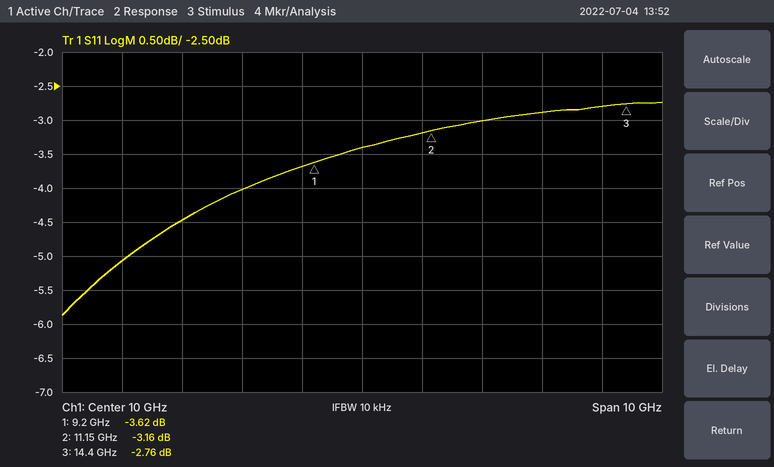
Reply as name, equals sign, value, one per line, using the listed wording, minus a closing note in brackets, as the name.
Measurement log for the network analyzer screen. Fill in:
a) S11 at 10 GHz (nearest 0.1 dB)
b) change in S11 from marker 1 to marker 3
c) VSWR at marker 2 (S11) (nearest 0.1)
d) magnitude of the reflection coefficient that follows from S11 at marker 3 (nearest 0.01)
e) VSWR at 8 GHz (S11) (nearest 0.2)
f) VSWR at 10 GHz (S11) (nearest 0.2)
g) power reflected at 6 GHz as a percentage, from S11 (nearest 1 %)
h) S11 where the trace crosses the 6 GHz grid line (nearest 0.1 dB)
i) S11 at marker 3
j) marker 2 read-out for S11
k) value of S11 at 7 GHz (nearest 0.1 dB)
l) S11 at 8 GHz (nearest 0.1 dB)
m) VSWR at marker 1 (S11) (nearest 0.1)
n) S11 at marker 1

S11 at 10 GHz = -3.4 dB
change in S11 from marker 1 to marker 3 = 0.86 dB
VSWR at marker 2 (S11) = 5.6
magnitude of the reflection coefficient that follows from S11 at marker 3 = 0.73
VSWR at 8 GHz (S11) = 4.4
VSWR at 10 GHz (S11) = 5.2
power reflected at 6 GHz as a percentage, from S11 = 31 %
S11 where the trace crosses the 6 GHz grid line = -5.1 dB
S11 at marker 3 = -2.76 dB
marker 2 read-out for S11 = -3.16 dB
value of S11 at 7 GHz = -4.5 dB
S11 at 8 GHz = -4.0 dB
VSWR at marker 1 (S11) = 4.9
S11 at marker 1 = -3.62 dB
